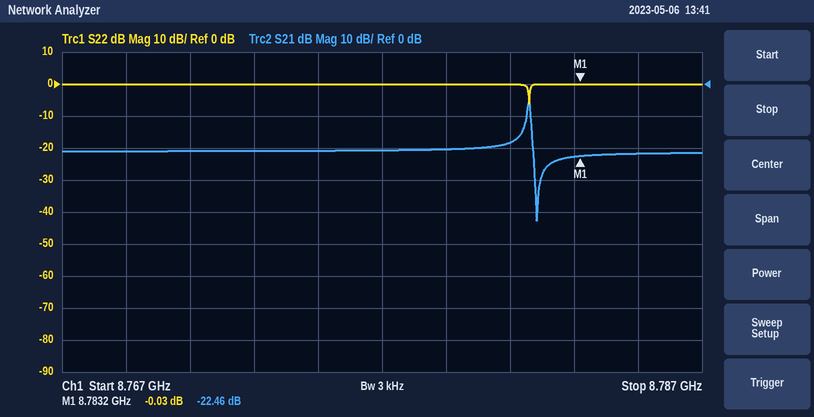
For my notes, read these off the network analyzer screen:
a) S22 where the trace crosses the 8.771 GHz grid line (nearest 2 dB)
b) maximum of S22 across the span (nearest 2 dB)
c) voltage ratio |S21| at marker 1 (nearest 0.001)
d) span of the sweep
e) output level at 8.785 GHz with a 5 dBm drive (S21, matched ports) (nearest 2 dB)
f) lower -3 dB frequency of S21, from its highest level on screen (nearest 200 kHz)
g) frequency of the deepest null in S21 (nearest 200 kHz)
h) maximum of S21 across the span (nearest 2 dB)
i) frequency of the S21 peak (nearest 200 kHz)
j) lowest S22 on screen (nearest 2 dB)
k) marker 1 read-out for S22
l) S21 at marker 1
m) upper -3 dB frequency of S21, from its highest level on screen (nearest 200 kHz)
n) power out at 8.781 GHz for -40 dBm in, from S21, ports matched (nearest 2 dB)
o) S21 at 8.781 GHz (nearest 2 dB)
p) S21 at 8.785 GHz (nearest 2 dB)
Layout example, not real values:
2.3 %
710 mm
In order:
0 dB
0 dB
0.075
20 MHz
-16 dBm
8.7816 GHz
8.7818 GHz
-6 dB
8.7816 GHz
-6 dB
-0.03 dB
-22.46 dB
8.7816 GHz
-58 dBm
-18 dB
-22 dB
